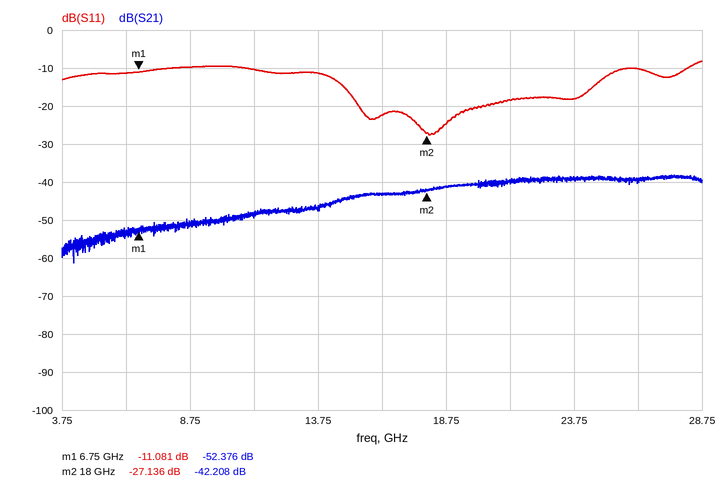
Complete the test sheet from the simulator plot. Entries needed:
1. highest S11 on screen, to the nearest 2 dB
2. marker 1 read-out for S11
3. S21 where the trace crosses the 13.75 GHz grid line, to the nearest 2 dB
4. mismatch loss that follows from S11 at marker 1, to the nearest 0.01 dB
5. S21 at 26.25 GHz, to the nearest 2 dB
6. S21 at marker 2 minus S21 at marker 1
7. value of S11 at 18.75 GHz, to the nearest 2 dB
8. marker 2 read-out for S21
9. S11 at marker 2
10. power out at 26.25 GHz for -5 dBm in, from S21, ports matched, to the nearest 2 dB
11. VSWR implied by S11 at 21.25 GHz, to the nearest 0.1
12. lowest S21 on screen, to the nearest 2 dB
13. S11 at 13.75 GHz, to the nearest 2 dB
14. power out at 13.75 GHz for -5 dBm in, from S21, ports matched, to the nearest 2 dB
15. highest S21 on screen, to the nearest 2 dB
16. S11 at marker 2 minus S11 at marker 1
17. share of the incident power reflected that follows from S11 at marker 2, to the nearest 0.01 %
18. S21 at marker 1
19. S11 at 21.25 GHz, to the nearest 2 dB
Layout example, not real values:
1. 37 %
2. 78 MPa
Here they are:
1. -8 dB
2. -11.081 dB
3. -46 dB
4. 0.35 dB
5. -40 dB
6. 10.168 dB
7. -24 dB
8. -42.208 dB
9. -27.136 dB
10. -44 dBm
11. 1.3
12. -62 dB
13. -12 dB
14. -52 dBm
15. -38 dB
16. -16.055 dB
17. 0.19 %
18. -52.376 dB
19. -18 dB
